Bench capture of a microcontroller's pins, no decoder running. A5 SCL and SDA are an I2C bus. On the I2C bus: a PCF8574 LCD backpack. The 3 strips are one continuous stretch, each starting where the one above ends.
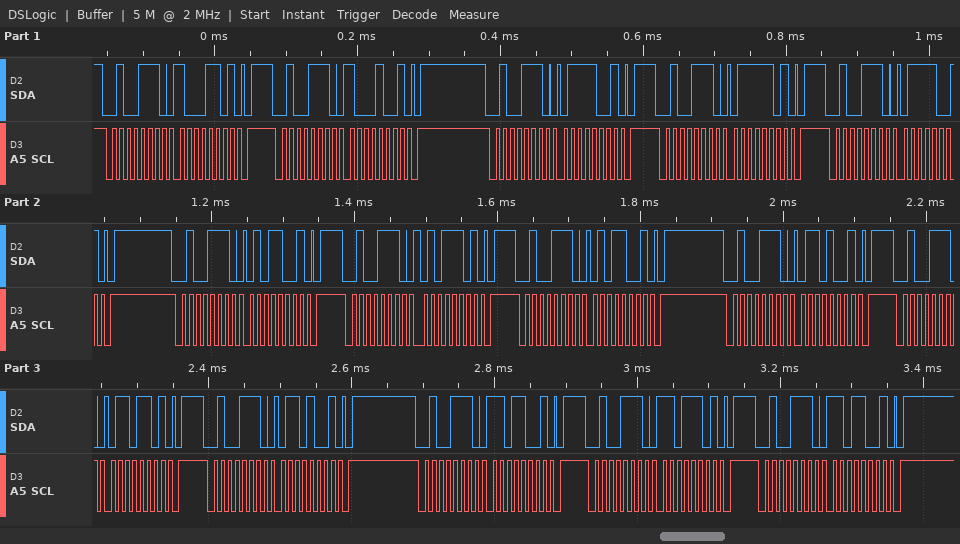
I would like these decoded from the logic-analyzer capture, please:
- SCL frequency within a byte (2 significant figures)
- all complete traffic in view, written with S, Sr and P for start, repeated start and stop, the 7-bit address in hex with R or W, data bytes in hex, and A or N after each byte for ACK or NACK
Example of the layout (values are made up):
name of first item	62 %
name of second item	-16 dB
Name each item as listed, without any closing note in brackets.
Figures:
SCL frequency within a byte	100 kHz
all complete traffic in view, written with S, Sr and P for start, repeated start and stop, the 7-bit address in hex with R or W, data bytes in hex, and A or N after each byte for ACK or NACK	S 27W A 8D A P S 27W A 89 A P S 27W A 79 A P S 27W A 7D A P S 27W A 79 A P S 27W A 59 A P S 27W A 5D A P S 27W A 59 A P S 27W A 69 A P S 27W A 6D A P S 27W A 69 A P S 27W A D9 A P S 27W A DD A P S 27W A D9 A P
